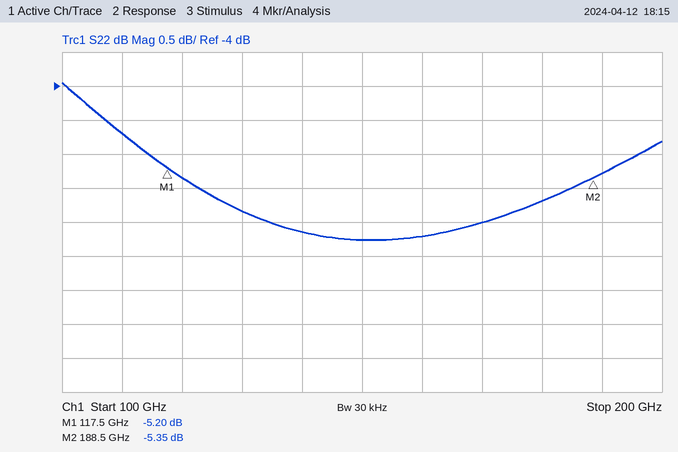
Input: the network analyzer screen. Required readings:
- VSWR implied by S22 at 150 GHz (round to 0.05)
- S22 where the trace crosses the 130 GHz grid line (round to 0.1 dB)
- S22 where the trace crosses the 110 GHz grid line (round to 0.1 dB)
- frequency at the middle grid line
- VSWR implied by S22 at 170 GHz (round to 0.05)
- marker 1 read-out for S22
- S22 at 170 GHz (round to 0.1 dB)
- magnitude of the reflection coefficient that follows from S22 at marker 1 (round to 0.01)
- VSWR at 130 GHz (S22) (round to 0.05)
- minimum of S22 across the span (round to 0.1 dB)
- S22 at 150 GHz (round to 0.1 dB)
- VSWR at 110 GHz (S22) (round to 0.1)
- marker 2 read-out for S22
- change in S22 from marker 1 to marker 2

2.90
-5.8 dB
-4.7 dB
150 GHz
3.00
-5.20 dB
-6.0 dB
0.55
3.10
-6.3 dB
-6.3 dB
3.8
-5.35 dB
-0.15 dB
